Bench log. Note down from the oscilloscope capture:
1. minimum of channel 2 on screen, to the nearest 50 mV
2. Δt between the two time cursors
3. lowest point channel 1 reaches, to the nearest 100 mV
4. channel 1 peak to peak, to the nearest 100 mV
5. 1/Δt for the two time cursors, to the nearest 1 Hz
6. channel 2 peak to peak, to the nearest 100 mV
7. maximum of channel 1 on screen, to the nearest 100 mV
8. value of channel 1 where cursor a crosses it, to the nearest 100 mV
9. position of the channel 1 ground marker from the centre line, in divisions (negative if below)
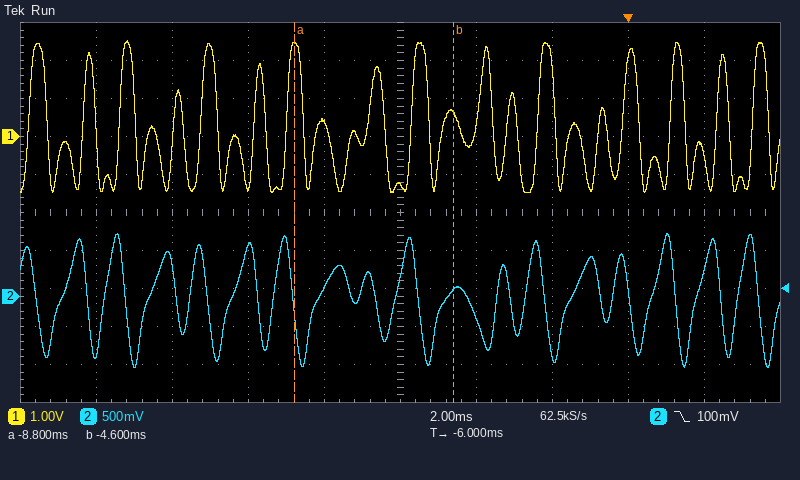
-950 mV
4.2 ms
-1.5 V
4.0 V
238 Hz
1.80 V
2.5 V
2.4 V
+2.0 div
